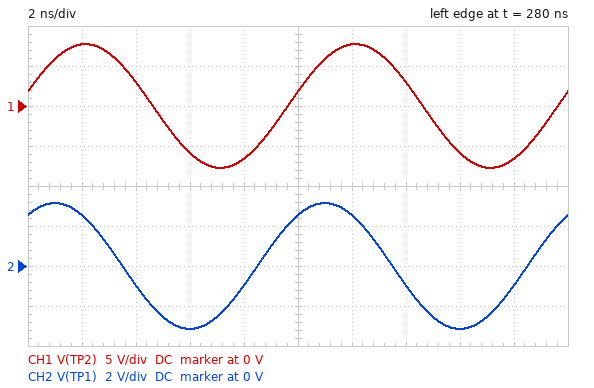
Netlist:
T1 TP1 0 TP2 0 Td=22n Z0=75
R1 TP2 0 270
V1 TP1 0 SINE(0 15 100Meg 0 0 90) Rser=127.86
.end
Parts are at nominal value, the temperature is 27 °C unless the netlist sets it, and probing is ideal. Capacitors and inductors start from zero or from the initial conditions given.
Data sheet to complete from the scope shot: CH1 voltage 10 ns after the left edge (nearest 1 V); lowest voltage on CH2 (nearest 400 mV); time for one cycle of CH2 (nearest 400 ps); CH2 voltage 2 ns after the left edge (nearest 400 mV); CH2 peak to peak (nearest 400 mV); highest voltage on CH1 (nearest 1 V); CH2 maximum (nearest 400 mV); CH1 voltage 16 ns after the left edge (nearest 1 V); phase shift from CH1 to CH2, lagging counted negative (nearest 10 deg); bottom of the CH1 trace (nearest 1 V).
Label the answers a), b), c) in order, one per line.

a) 2 V
b) -3.2 V
c) 10.0 ns
d) 2.4 V
e) 6.4 V
f) 8 V
g) 3.2 V
h) -6 V
i) 40 deg
j) -8 V
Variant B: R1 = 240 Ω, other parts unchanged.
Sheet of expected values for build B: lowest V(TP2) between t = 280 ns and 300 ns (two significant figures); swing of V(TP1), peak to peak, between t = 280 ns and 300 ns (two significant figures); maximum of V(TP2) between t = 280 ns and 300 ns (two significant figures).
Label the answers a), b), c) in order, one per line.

a) -7.6 V
b) 6.5 V
c) 7.6 V
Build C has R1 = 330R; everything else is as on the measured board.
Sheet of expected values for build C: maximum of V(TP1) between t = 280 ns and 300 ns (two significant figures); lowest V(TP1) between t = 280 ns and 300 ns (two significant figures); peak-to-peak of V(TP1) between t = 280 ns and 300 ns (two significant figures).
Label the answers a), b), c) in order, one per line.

a) 3.0 V
b) -3.0 V
c) 6.0 V
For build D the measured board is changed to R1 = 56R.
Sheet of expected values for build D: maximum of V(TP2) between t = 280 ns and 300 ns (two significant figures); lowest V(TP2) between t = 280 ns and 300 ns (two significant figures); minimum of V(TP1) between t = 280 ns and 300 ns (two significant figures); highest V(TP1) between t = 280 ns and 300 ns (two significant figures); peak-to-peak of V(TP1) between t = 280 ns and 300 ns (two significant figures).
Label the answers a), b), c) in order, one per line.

a) 4.9 V
b) -4.9 V
c) -6.4 V
d) 6.4 V
e) 13 V
